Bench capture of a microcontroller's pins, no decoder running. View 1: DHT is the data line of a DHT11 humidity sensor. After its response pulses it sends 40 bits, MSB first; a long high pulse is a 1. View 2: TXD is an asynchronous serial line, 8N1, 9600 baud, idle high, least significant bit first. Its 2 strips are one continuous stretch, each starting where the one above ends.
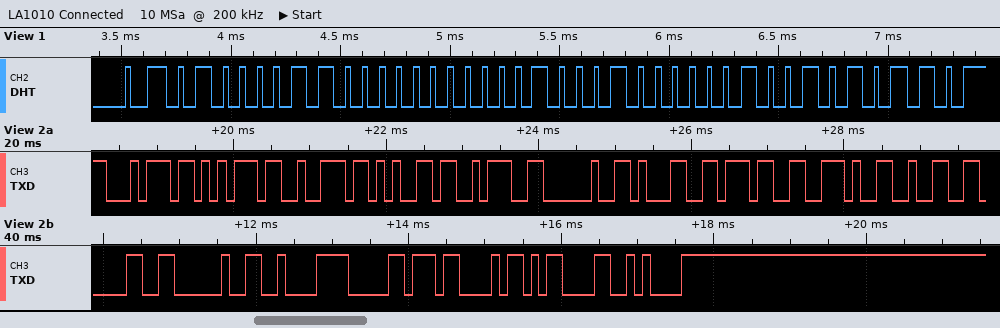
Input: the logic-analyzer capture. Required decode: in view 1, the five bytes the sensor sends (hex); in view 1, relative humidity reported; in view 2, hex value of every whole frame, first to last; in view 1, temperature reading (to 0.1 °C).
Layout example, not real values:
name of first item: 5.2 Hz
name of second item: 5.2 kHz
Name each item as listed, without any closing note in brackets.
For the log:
in view 1, the five bytes the sensor sends: 43 00 11 02 56
in view 1, relative humidity reported: 67 %
in view 2, hex value of every whole frame, first to last: 74 75 72 65 3A 20 31 37 2E 32 30 20 C2 B0 43 0D 0A
in view 1, temperature reading: 17.2 °C
